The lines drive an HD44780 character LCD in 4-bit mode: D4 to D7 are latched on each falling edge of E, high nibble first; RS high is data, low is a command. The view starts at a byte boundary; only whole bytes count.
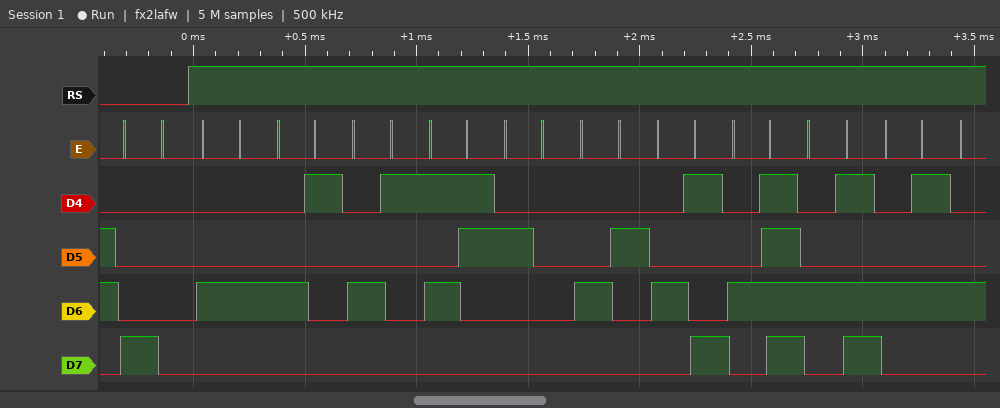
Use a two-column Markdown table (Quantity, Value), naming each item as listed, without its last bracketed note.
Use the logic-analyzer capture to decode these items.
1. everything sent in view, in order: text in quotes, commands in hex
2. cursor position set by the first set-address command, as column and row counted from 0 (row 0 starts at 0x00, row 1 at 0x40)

| Quantity | Value |
|---|---|
| everything sent in view, in order: text in quotes, commands in hex | 0x80 "DAAS BIOME" |
| cursor position set by the first set-address command, as column and row counted from 0 | column 0, row 0 |
